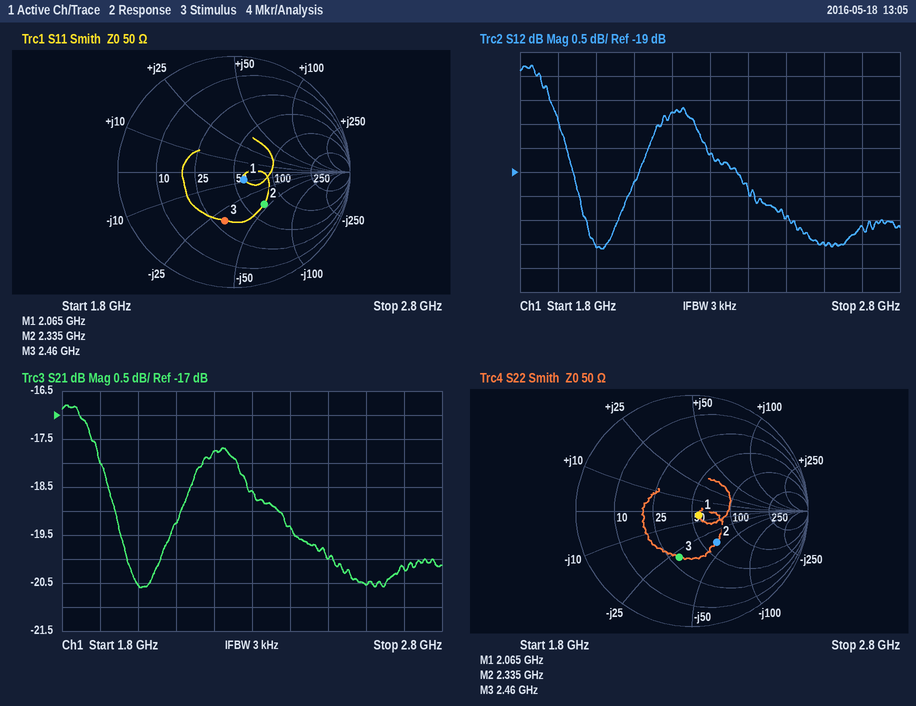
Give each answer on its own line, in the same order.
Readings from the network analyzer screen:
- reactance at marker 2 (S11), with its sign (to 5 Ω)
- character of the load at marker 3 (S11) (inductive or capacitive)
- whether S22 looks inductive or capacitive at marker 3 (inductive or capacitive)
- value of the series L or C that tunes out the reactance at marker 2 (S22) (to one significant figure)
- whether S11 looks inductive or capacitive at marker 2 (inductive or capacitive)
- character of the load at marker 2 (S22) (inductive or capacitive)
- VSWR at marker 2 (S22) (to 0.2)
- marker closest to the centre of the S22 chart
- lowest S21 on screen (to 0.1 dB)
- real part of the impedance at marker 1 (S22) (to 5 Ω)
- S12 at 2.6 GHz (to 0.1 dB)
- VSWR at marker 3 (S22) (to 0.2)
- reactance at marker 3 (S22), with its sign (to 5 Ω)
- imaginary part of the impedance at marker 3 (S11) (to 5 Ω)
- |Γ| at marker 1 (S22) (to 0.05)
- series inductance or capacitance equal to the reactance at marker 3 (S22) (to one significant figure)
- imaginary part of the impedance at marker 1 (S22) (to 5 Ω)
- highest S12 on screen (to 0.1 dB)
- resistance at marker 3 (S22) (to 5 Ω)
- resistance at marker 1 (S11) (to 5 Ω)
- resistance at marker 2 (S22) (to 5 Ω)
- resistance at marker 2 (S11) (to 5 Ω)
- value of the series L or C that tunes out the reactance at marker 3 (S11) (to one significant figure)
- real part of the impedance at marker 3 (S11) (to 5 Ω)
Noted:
-45 Ω
capacitive
capacitive
3 nH
capacitive
capacitive
2.0
marker 1
-20.6 dB
55 Ω
-20.5 dB
2.4
-30 Ω
-30 Ω
0.05
2 pF
-5 Ω
-16.8 dB
30 Ω
60 Ω
65 Ω
70 Ω
2 nH
30 Ω
